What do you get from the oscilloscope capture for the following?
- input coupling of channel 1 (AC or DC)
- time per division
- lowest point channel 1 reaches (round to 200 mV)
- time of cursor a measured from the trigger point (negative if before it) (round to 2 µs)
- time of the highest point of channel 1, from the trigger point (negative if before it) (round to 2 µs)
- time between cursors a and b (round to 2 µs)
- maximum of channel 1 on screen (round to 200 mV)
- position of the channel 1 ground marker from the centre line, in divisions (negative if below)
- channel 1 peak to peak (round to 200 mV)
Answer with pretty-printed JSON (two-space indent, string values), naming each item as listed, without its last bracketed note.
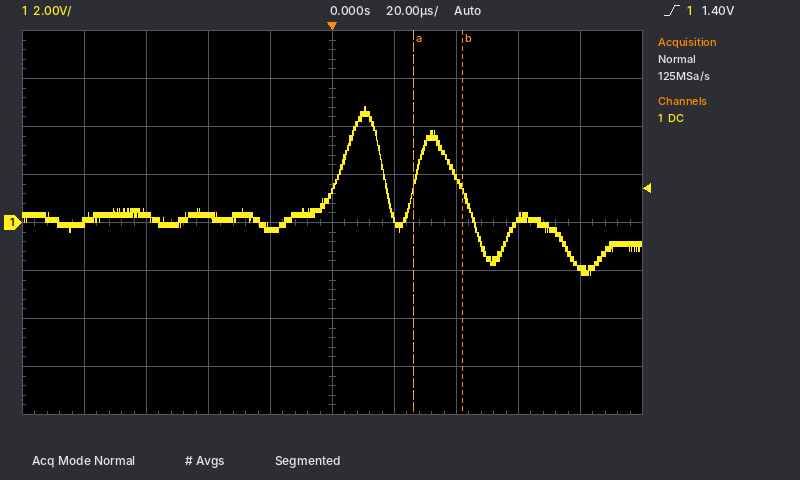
{
  "input coupling of channel 1": "DC",
  "time per division": "20 µs",
  "lowest point channel 1 reaches": "-2.2 V",
  "time of cursor a measured from the trigger point (negative if before it)": "+26 µs",
  "time of the highest point of channel 1, from the trigger point (negative if before it)": "+10 µs",
  "time between cursors a and b": "16 µs",
  "maximum of channel 1 on screen": "4.8 V",
  "position of the channel 1 ground marker from the centre line, in divisions": "0.0 div",
  "channel 1 peak to peak": "7.0 V"
}
